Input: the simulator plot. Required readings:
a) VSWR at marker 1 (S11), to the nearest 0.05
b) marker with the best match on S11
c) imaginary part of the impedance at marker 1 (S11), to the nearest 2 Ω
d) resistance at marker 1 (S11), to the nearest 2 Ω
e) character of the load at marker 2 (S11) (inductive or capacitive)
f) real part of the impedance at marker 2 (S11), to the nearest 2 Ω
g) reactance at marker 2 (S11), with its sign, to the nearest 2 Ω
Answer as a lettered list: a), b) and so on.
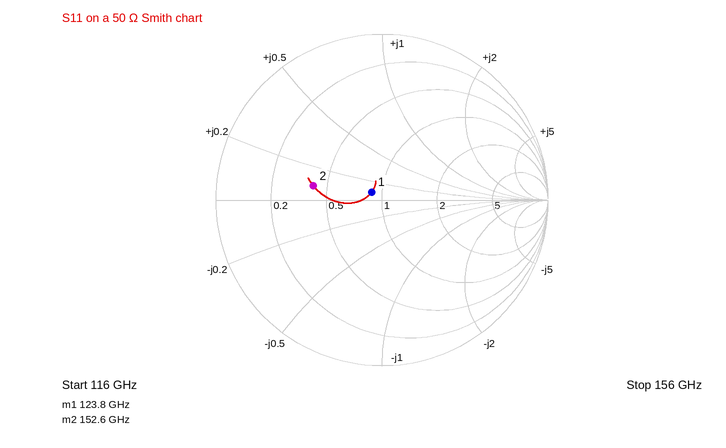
a) 1.15
b) marker 1
c) +4 Ω
d) 44 Ω
e) inductive
f) 20 Ω
g) +4 Ω
